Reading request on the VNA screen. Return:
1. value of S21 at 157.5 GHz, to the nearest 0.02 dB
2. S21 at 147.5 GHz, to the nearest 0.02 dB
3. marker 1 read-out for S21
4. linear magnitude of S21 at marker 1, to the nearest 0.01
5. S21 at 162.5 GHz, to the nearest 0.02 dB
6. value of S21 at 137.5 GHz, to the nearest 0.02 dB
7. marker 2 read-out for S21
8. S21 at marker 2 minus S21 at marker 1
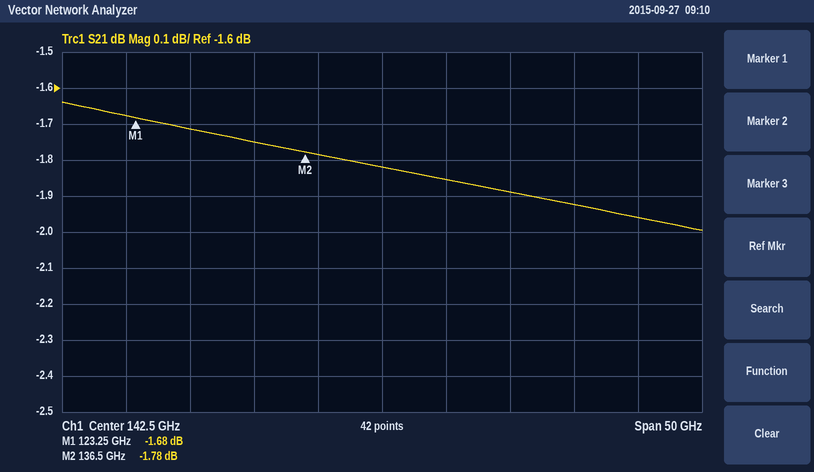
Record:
-1.92 dB
-1.86 dB
-1.68 dB
0.82
-1.96 dB
-1.78 dB
-1.78 dB
-0.10 dB
